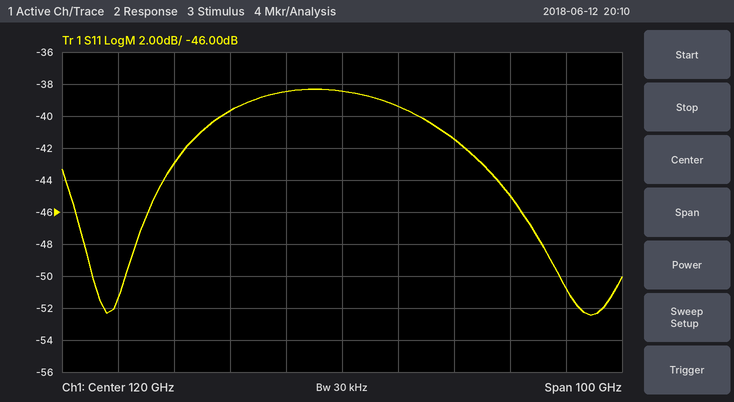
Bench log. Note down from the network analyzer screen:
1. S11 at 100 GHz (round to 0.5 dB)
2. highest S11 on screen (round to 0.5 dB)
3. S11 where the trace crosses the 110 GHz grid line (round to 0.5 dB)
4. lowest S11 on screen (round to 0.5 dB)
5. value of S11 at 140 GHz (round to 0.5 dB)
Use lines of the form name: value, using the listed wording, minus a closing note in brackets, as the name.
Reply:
S11 at 100 GHz: -39.5 dB
highest S11 on screen: -38.5 dB
S11 where the trace crosses the 110 GHz grid line: -38.5 dB
lowest S11 on screen: -52.5 dB
value of S11 at 140 GHz: -41.5 dB
